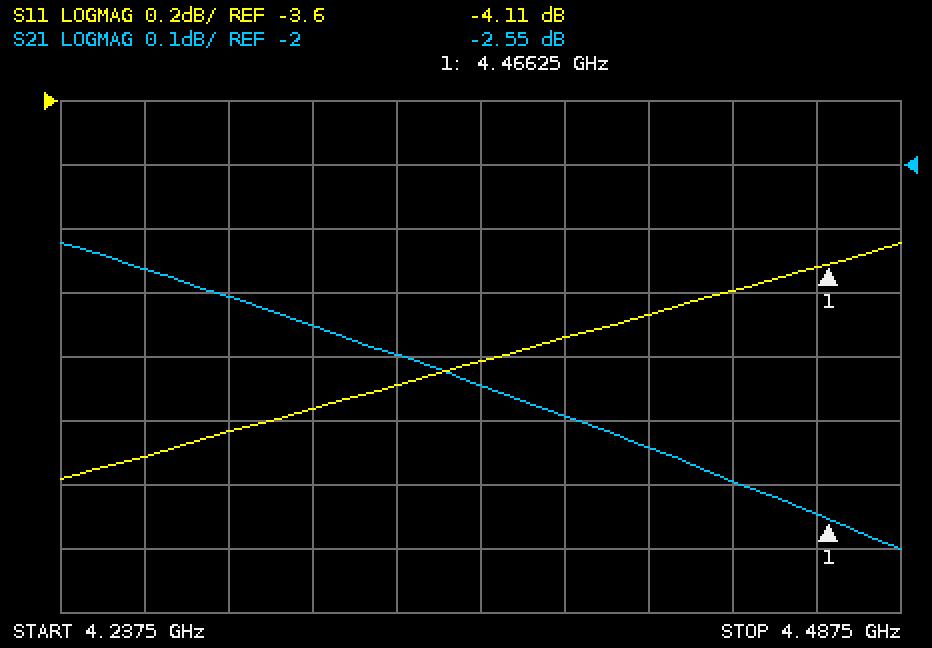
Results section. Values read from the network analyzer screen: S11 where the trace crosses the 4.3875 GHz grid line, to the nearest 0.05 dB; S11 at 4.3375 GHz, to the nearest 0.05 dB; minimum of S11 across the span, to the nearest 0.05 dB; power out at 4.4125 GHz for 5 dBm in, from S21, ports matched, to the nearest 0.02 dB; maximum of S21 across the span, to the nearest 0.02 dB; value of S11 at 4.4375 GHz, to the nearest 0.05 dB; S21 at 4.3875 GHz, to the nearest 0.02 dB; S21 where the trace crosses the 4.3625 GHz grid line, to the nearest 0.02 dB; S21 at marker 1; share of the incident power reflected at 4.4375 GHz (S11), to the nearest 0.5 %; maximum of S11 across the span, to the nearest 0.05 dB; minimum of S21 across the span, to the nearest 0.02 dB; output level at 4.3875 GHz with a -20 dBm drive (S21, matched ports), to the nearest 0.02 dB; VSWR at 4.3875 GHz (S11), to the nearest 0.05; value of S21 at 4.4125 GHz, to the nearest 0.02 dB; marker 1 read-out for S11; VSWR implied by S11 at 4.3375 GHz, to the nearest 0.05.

-4.35 dB
-4.50 dB
-4.80 dB
2.56 dBm
-2.12 dB
-4.20 dB
-2.40 dB
-2.34 dB
-2.55 dB
38.0 %
-4.05 dB
-2.60 dB
-22.40 dBm
4.10
-2.44 dB
-4.11 dB
3.95
